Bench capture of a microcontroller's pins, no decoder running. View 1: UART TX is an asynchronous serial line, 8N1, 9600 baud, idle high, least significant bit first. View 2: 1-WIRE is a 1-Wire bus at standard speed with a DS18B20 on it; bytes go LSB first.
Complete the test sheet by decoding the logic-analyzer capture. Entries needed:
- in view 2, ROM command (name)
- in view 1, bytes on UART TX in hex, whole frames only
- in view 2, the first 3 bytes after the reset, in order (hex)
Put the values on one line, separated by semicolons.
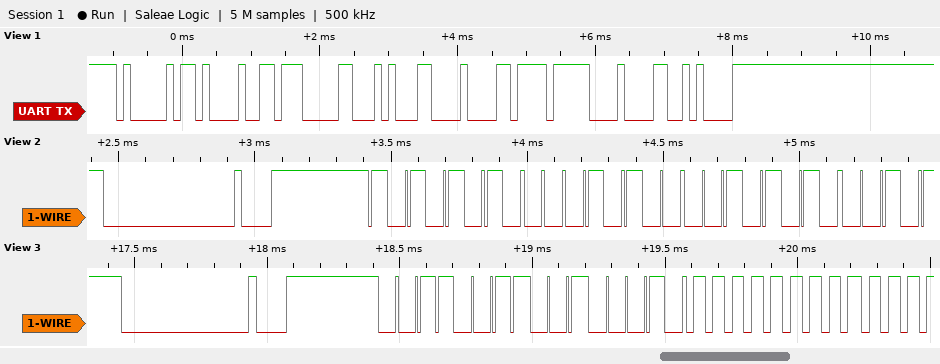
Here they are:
Match ROM; 41 21 07 14 08 EF 08 0A; 55 28 54
